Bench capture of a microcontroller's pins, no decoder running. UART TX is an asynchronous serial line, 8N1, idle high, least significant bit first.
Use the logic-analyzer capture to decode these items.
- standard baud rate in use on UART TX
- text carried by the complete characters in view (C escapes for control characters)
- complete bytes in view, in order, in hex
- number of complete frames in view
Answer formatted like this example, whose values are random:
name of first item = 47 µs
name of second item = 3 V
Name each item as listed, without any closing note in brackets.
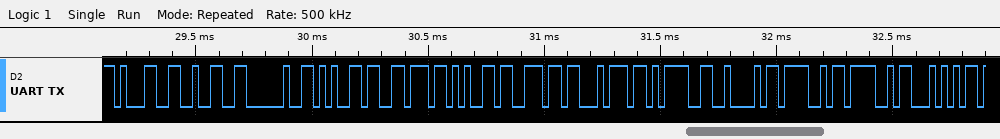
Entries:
standard baud rate in use on UART TX = 38400 baud
text carried by the complete characters in view = "12 event=BOOT"
complete bytes in view, in order, in hex = 0x31 0x32 0x20 0x65 0x76 0x65 0x6E 0x74 0x3D 0x42 0x4F 0x4F 0x54
number of complete frames in view = 13
